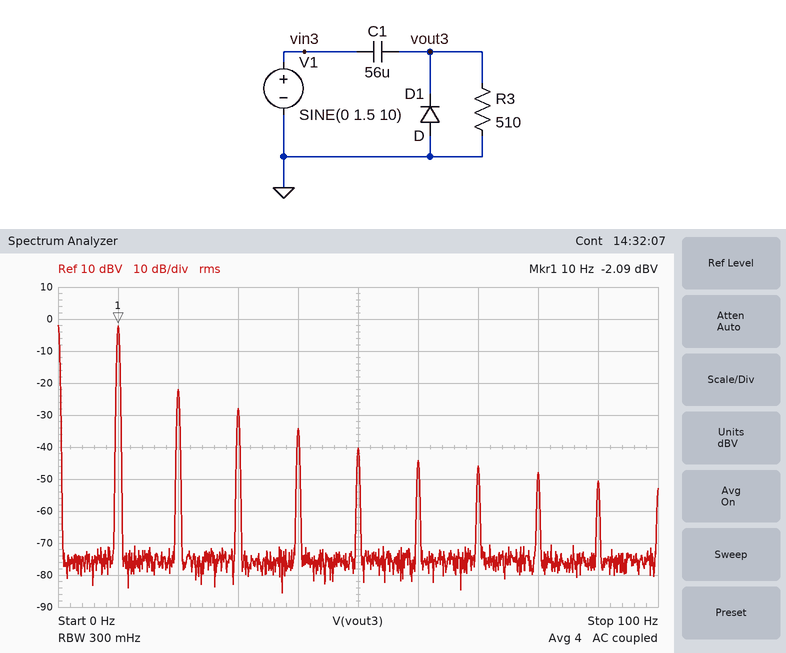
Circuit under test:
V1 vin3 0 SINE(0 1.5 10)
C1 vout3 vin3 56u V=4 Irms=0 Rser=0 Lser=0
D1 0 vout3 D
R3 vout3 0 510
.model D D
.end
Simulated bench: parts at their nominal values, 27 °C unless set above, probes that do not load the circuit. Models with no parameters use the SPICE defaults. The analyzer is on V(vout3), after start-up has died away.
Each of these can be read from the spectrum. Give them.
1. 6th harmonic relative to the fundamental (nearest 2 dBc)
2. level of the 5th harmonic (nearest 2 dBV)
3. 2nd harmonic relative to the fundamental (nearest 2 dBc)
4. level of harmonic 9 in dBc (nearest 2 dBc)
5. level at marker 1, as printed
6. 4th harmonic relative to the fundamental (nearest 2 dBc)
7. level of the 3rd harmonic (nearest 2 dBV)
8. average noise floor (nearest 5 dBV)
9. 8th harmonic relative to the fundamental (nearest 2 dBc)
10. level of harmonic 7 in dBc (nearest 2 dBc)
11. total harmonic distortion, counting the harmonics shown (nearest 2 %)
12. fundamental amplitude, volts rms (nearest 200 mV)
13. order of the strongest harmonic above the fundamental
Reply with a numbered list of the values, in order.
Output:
1. -42 dBc
2. -40 dBV
3. -20 dBc
4. -48 dBc
5. -2.09 dBV
6. -32 dBc
7. -28 dBV
8. -75 dBV
9. -46 dBc
10. -44 dBc
11. 12 %
12. 800 mV
13. 2
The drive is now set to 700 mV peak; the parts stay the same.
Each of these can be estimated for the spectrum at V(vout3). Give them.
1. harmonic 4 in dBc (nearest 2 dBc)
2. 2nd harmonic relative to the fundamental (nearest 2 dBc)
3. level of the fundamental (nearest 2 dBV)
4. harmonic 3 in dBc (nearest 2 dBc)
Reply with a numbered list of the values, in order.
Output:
1. -56 dBc
2. -48 dBc
3. -8 dBV
4. -52 dBc
